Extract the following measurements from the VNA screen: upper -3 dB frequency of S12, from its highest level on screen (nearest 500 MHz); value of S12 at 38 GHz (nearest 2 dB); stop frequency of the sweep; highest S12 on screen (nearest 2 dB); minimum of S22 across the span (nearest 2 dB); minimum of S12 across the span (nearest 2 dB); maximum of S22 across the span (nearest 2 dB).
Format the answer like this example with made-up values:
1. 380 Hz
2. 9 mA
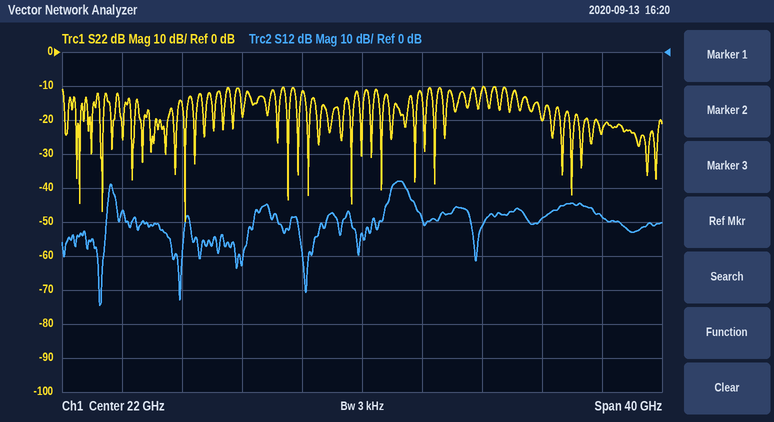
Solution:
1. 25.0 GHz
2. -48 dB
3. 42 GHz
4. -38 dB
5. -50 dB
6. -74 dB
7. -10 dB
